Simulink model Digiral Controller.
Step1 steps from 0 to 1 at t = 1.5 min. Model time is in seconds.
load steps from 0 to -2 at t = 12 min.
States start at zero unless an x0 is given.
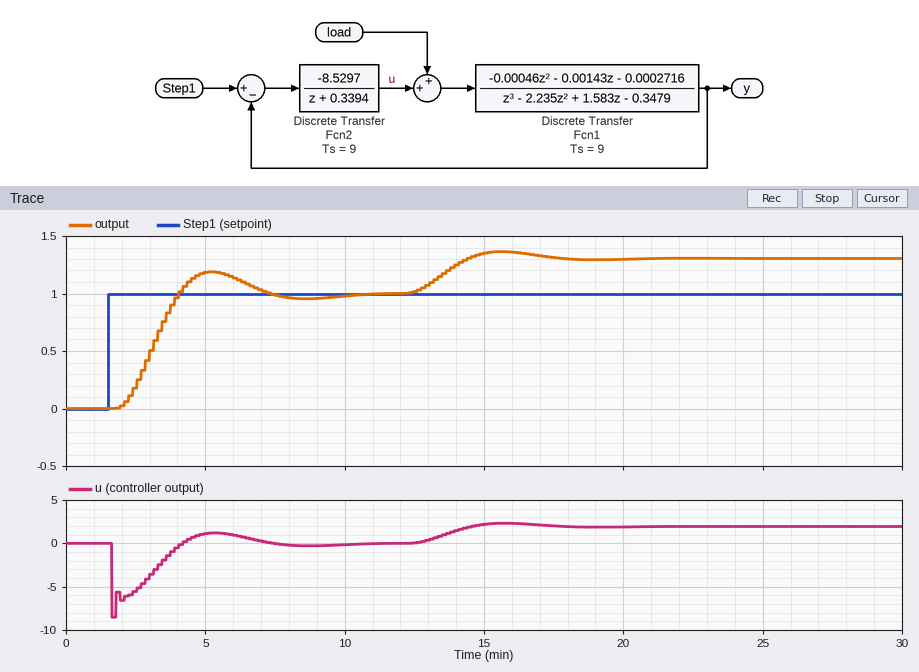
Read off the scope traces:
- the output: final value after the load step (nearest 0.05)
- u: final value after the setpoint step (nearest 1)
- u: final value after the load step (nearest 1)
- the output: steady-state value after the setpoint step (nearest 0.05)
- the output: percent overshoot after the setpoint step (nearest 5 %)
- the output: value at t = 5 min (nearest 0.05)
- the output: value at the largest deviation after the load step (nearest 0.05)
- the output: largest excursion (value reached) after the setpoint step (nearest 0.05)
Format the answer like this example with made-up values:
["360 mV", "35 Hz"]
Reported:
["1.30", "0", "2", "1.00", "20 %", "1.20", "1.35", "1.20"]
